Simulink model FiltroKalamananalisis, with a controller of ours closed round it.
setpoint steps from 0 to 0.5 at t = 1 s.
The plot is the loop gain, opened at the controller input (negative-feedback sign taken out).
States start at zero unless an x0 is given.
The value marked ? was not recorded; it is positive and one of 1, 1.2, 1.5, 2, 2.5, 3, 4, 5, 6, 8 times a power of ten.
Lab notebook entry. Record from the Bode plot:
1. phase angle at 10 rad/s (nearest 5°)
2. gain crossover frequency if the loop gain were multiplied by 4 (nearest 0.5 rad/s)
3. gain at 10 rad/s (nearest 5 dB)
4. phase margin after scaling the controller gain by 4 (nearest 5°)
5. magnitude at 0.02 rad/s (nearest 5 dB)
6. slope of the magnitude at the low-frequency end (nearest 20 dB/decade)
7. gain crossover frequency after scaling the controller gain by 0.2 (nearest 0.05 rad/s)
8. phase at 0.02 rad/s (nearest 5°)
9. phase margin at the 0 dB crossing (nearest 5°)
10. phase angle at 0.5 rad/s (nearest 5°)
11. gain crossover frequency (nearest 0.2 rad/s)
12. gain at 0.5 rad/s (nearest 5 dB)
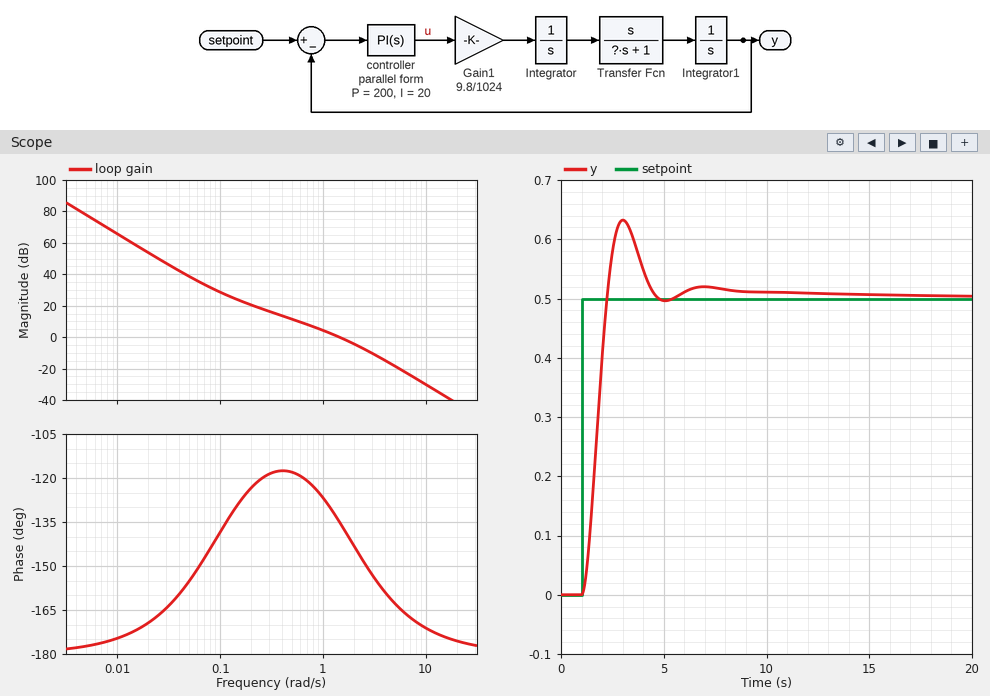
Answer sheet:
-170°
3.5 rad/s
-30 dB
25°
55 dB
-40 dB/decade
0.40 rad/s
-170°
45°
-120°
1.4 rad/s
10 dB
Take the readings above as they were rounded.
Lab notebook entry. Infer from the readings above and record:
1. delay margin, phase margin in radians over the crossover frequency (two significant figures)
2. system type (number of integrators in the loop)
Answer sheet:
0.56 s
2
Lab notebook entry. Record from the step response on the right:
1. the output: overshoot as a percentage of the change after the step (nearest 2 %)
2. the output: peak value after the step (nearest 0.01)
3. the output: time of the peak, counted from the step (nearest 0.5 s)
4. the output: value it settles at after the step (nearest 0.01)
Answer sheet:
26 %
0.63
2.0 s
0.50
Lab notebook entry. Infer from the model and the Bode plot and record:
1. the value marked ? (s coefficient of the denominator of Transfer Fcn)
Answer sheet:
0.6
